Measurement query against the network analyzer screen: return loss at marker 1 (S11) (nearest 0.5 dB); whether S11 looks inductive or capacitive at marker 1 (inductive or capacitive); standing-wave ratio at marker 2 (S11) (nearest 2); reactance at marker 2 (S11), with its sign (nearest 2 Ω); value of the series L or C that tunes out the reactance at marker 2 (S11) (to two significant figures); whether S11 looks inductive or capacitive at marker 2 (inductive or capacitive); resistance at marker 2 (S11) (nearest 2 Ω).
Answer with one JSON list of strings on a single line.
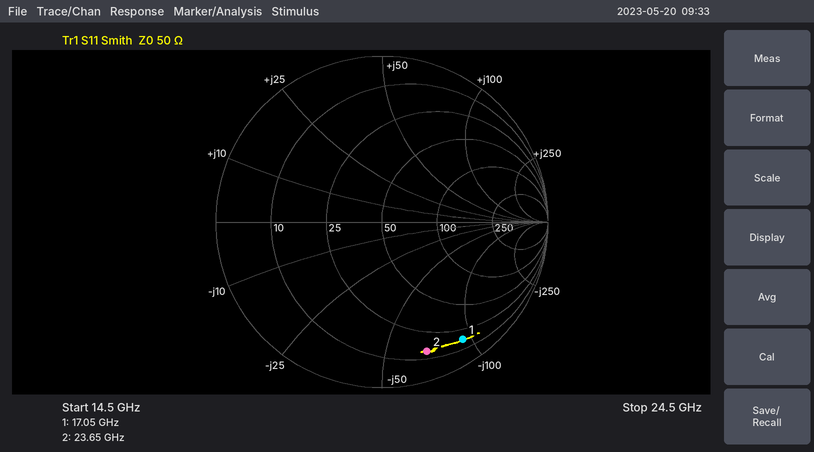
["1.5 dB", "capacitive", "10", "-68 Ω", "460 pH", "capacitive", "14 Ω"]
